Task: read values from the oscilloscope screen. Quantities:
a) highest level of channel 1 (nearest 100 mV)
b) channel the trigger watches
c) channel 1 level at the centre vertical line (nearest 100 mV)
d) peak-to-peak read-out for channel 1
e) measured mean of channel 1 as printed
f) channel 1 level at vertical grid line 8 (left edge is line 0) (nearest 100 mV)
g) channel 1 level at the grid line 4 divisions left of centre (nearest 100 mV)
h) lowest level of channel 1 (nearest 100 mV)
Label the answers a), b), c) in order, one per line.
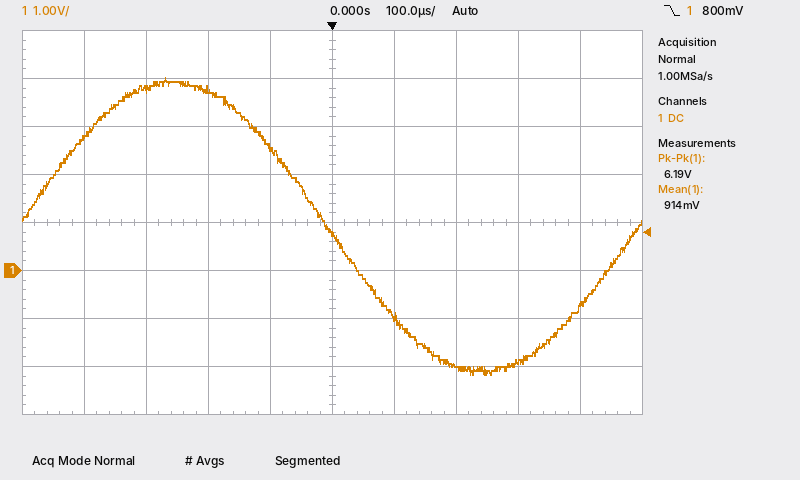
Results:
a) 4.0 V
b) channel 1
c) 800 mV
d) 6.19 V
e) 914 mV
f) -1.9 V
g) 2.8 V
h) -2.2 V
